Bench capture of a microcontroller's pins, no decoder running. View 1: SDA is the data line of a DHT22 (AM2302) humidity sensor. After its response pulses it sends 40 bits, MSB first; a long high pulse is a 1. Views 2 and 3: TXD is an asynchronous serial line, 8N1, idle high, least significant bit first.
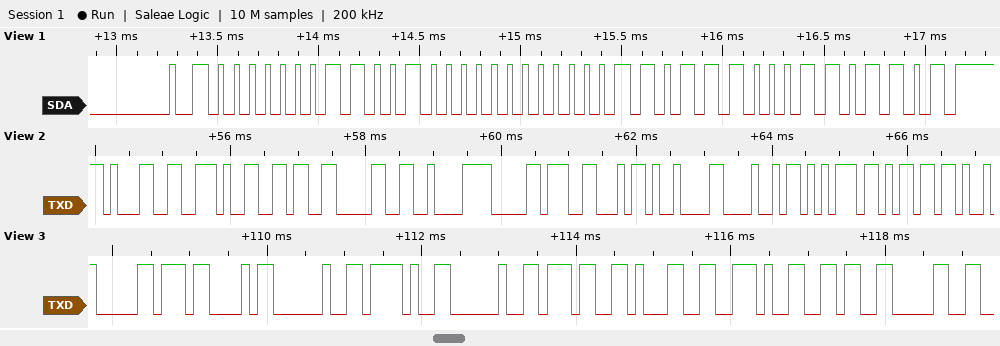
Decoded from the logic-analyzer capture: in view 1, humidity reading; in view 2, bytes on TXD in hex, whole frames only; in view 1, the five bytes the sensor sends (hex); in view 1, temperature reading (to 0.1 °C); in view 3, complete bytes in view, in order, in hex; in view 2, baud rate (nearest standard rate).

40.0 %
0x31 0x2E 0x36 0x30 0xC2 0xB0 0x46 0x09 0x48 0x75 0x6D
01 90 00 DC 6D
22.0 °C
0xB0 0x43 0x20 0x2F 0x20 0x37 0x31 0x2E 0x36 0x30
9600 baud
